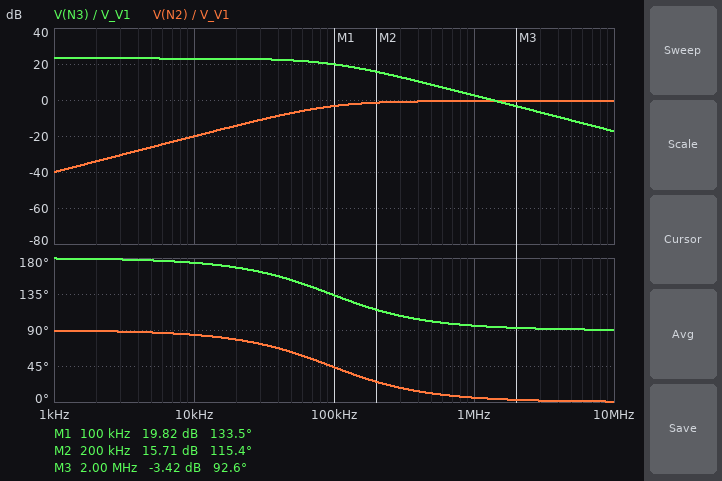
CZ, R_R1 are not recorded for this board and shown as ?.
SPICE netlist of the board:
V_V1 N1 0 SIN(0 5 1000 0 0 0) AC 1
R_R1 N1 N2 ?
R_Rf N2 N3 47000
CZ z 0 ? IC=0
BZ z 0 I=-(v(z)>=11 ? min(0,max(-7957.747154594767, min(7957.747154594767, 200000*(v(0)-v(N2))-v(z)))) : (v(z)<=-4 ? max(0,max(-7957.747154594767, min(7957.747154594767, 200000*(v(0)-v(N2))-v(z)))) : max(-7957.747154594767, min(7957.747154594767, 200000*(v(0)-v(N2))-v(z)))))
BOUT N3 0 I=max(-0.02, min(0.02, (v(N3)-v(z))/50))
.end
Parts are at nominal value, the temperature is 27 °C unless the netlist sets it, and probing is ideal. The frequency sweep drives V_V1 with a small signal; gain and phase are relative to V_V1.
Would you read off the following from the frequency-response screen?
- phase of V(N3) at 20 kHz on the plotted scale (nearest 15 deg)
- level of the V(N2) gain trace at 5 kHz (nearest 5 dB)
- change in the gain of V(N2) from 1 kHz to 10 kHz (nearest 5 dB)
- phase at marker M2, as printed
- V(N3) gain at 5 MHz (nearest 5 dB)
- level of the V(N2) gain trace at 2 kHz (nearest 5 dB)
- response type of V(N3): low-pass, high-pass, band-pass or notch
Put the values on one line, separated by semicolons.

165 deg; -25 dB; 20 dB; 115.4 deg; -10 dB; -35 dB; low-pass
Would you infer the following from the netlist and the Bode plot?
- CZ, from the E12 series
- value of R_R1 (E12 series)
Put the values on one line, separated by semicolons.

22 mF; 3.3 kΩ
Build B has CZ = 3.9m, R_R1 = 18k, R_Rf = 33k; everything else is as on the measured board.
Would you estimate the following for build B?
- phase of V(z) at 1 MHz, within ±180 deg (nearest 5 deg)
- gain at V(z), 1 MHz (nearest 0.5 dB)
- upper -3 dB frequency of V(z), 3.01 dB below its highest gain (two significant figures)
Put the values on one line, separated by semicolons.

160 deg; 5.0 dB; 2.9 MHz
